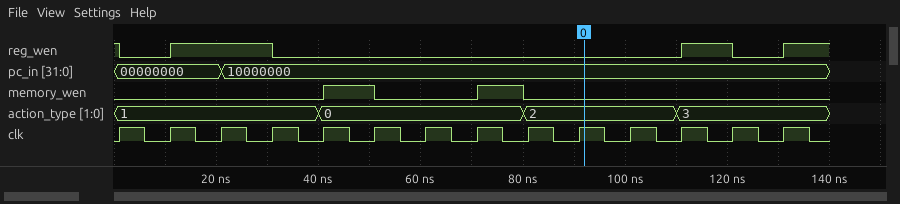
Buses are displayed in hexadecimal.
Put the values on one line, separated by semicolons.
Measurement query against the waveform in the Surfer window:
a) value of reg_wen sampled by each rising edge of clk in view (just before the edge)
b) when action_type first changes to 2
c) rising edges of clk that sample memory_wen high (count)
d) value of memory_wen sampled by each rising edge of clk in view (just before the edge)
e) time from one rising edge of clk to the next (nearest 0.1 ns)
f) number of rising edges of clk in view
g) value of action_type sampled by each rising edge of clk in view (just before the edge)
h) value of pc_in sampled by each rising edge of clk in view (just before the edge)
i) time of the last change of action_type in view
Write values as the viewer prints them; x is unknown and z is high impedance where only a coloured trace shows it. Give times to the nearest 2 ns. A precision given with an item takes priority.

1 0 1 1 0 0 0 0 0 0 0 0 1 0; 80 ns; 1; 0 0 0 0 0 1 0 0 0 0 0 0 0 0; 10 ns; 14; 1, 1, 1, 1, 0, 0, 0, 0, 2, 2, 2, 3, 3, 3; 00000000, 00000000, 00000000, 10000000, 10000000, 10000000, 10000000, 10000000, 10000000, 10000000, 10000000, 10000000, 10000000, 10000000; 110 ns
